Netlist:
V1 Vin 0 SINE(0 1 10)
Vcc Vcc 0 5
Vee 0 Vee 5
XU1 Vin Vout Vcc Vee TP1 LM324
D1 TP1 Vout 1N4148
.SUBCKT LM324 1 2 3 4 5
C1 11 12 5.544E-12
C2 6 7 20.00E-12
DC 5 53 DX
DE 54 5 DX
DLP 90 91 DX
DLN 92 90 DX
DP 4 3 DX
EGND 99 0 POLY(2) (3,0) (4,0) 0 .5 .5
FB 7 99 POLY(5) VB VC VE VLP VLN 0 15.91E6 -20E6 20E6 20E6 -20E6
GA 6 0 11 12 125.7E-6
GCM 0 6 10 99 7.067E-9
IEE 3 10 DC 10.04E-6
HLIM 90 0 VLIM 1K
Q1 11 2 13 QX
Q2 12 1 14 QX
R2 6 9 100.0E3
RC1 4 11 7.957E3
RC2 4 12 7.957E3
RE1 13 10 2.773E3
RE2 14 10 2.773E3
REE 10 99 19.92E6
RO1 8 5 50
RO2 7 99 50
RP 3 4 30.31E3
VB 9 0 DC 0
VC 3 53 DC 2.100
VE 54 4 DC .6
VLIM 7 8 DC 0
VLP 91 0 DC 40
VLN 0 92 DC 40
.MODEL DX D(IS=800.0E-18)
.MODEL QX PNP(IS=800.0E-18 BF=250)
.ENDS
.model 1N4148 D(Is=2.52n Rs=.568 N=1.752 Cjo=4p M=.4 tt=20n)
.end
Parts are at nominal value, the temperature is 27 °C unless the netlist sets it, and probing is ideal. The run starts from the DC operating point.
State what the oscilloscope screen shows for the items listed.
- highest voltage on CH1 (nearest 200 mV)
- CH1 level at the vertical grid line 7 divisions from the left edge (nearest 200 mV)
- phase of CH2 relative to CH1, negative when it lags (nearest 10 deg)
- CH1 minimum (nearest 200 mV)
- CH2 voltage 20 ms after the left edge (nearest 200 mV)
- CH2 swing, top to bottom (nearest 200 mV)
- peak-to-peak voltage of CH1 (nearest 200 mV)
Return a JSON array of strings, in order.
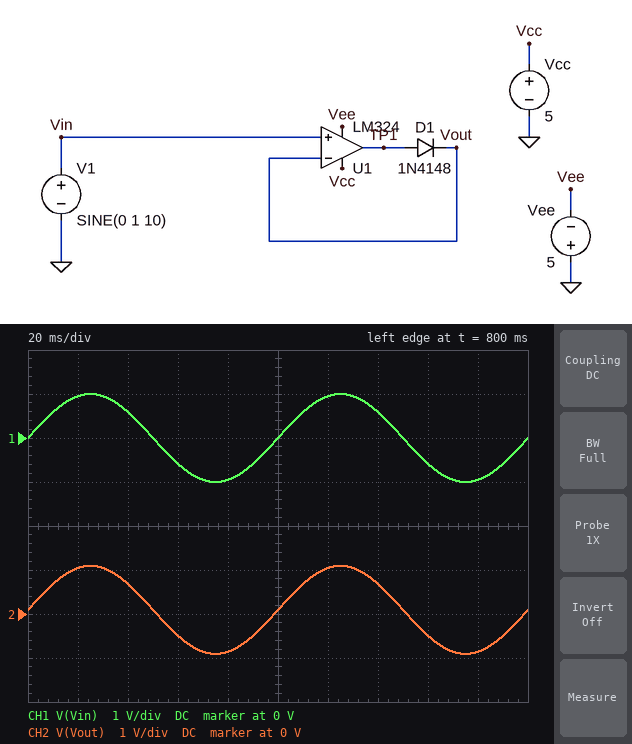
["1.0 V", "600 mV", "0 deg", "-1.0 V", "1.0 V", "2.0 V", "2.0 V"]
